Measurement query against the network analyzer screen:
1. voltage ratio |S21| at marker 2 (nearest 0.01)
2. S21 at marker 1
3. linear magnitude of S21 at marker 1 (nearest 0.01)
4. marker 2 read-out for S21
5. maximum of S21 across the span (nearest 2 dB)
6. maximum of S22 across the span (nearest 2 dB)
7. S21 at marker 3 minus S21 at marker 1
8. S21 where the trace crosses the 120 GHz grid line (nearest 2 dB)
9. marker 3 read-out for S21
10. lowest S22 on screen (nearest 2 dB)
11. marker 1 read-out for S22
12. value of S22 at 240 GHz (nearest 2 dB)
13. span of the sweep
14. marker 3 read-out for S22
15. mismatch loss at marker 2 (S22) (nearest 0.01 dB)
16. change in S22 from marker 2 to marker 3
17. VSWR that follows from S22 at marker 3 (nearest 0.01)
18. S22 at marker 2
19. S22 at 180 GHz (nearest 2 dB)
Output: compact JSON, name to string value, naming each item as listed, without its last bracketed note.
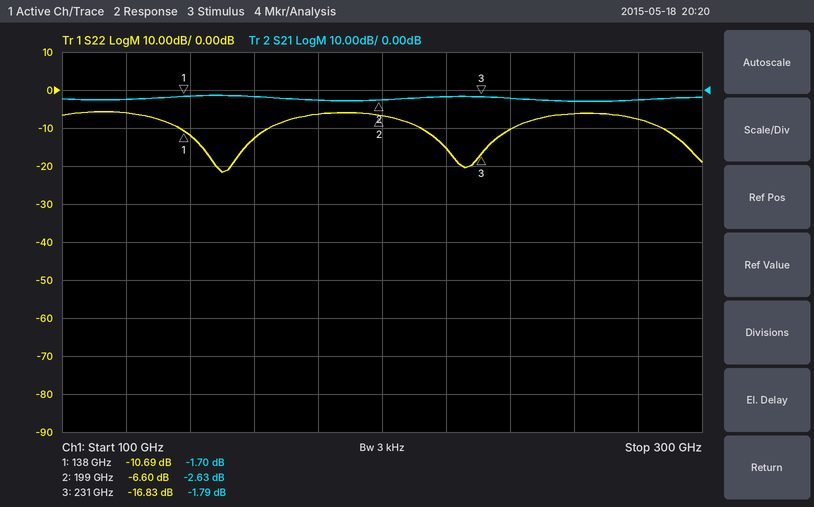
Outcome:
{"voltage ratio |S21| at marker 2": "0.74", "S21 at marker 1": "-1.70 dB", "linear magnitude of S21 at marker 1": "0.82", "marker 2 read-out for S21": "-2.63 dB", "maximum of S21 across the span": "-2 dB", "maximum of S22 across the span": "-6 dB", "S21 at marker 3 minus S21 at marker 1": "-0.09 dB", "S21 where the trace crosses the 120 GHz grid line": "-2 dB", "marker 3 read-out for S21": "-1.79 dB", "lowest S22 on screen": "-22 dB", "marker 1 read-out for S22": "-10.69 dB", "value of S22 at 240 GHz": "-10 dB", "span of the sweep": "200 GHz", "marker 3 read-out for S22": "-16.83 dB", "mismatch loss at marker 2 (S22)": "1.07 dB", "change in S22 from marker 2 to marker 3": "-10.23 dB", "VSWR that follows from S22 at marker 3": "1.34", "S22 at marker 2": "-6.60 dB", "S22 at 180 GHz": "-6 dB"}
